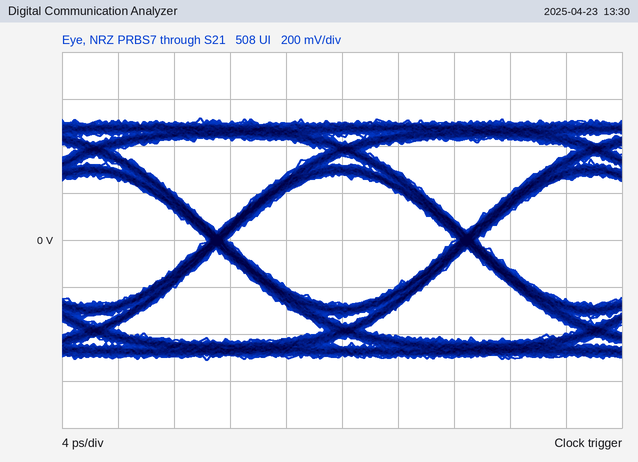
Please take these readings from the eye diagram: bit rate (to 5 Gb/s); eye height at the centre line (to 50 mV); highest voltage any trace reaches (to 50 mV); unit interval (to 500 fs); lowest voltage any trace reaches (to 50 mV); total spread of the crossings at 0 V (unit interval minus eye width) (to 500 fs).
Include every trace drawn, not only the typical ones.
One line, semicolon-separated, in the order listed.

55 Gb/s; 550 mV; 500 mV; 18.0 ps; -500 mV; 1.5 ps
